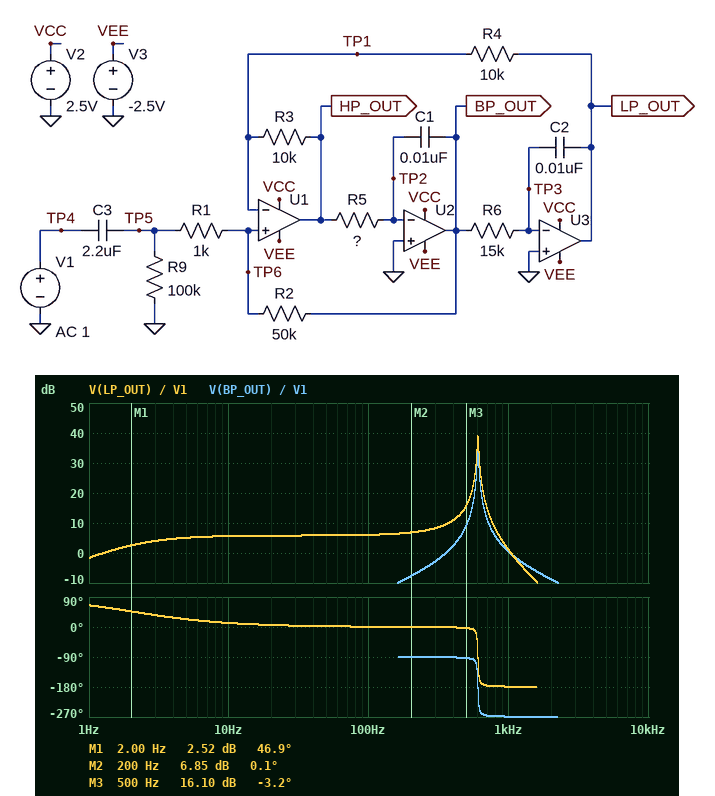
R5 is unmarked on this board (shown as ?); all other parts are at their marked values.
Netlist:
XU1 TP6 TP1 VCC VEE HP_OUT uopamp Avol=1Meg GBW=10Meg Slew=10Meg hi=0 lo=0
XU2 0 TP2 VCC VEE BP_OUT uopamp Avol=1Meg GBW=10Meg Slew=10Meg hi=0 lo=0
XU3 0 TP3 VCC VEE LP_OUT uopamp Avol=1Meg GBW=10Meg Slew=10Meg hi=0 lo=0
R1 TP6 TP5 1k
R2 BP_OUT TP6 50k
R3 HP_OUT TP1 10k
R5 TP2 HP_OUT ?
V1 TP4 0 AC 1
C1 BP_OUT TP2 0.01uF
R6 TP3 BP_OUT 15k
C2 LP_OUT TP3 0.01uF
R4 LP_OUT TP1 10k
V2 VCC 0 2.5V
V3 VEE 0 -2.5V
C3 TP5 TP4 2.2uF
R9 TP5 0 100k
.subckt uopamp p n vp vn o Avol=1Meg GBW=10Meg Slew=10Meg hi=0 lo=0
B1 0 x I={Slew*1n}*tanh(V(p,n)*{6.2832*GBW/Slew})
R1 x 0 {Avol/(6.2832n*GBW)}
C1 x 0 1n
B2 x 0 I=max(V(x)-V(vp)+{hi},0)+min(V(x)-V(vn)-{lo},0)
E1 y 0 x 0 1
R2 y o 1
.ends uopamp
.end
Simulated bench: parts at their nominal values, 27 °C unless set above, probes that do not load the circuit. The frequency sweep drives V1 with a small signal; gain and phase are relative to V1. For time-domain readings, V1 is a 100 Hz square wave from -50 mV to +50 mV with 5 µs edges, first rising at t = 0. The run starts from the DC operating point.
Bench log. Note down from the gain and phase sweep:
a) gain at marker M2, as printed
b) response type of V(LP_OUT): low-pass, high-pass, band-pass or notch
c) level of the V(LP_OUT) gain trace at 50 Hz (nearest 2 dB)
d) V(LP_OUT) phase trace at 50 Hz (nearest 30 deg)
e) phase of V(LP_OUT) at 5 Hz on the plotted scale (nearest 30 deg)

6.85 dB
band-pass
6 dB
0 deg
30 deg
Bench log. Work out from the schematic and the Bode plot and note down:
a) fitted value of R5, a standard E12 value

47 kΩ
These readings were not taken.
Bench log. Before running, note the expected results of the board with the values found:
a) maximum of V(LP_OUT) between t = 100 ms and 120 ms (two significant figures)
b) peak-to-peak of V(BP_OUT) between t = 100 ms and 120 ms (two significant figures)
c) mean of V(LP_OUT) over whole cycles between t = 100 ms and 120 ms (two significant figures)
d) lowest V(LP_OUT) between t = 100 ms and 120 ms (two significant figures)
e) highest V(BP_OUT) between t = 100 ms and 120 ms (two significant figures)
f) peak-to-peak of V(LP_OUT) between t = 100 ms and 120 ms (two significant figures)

230 mV
120 mV
38 mV
-180 mV
59 mV
410 mV
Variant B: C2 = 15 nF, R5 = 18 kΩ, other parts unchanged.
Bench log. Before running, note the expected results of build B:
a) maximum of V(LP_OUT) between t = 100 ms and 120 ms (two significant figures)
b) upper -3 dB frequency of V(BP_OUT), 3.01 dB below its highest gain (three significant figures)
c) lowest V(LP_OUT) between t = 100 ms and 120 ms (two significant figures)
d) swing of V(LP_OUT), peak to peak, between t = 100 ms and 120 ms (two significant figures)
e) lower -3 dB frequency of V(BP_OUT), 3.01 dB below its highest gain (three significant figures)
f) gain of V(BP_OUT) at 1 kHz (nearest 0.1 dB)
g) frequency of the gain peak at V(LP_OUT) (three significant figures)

240 mV
810 Hz
-200 mV
440 mV
775 Hz
13.3 dB
792 Hz
